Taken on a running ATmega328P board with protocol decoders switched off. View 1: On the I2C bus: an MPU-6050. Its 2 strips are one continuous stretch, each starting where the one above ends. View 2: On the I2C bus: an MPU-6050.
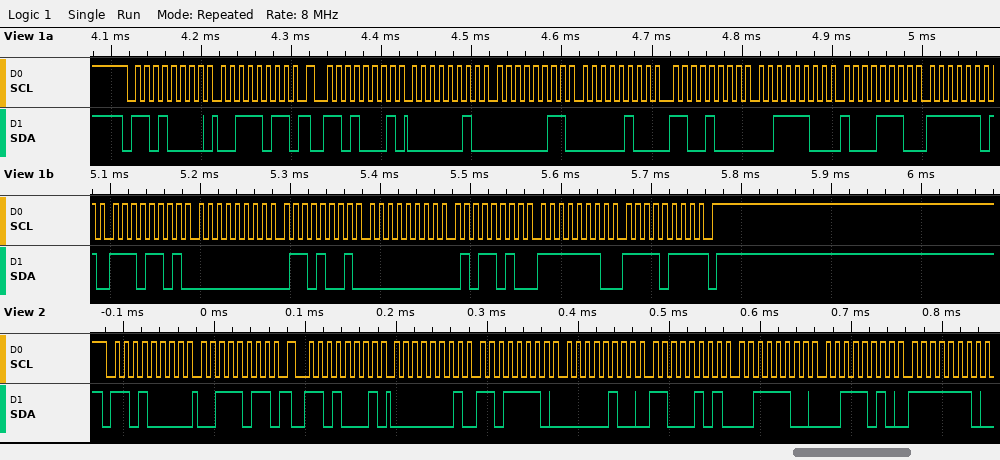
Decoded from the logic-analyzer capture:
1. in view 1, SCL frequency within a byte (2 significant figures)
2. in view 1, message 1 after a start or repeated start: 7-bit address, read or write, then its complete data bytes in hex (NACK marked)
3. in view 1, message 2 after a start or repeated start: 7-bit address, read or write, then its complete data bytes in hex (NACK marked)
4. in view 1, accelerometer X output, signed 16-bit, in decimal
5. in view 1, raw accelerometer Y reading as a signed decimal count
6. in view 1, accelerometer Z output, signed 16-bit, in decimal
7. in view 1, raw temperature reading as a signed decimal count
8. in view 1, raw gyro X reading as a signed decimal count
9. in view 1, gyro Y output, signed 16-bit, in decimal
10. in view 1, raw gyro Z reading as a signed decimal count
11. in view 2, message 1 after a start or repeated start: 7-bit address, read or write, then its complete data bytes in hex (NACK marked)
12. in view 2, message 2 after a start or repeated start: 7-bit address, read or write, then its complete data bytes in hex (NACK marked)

100 kHz
0x68 write: 3B
0x68 read: 02 03 04 C8 3C 8E FD ED 00 69 00 5A FE F7 NACK
515
1224
15502
-531
105
90
-265
0x68 write: 3B
0x68 read: 01 DE 04 C5 3C 3A FE
